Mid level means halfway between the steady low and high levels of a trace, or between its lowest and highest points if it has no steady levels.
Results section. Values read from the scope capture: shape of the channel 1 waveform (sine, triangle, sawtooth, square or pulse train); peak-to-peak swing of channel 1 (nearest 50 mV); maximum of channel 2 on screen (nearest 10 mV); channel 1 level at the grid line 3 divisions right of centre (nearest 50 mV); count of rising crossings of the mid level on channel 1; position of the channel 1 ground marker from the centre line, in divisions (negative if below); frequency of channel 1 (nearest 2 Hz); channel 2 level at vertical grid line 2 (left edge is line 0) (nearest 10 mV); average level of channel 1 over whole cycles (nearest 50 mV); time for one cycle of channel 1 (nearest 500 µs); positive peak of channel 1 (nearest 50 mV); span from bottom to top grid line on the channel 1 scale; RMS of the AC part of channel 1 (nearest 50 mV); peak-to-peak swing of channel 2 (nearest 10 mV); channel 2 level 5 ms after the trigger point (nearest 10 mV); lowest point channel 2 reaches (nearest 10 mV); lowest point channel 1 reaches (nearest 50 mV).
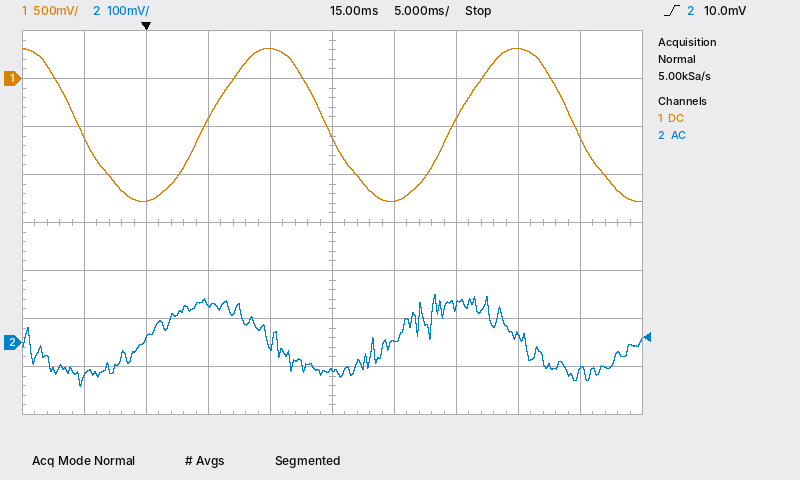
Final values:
sine
1.60 V
100 mV
300 mV
2
+3.0 div
50 Hz
10 mV
-500 mV
20.0 ms
300 mV
4 V
550 mV
190 mV
80 mV
-90 mV
-1.30 V
